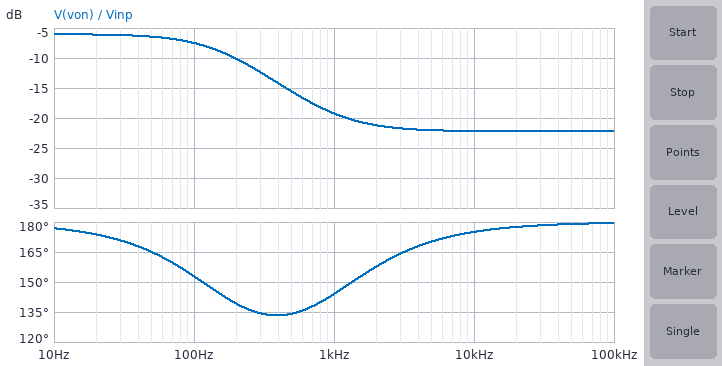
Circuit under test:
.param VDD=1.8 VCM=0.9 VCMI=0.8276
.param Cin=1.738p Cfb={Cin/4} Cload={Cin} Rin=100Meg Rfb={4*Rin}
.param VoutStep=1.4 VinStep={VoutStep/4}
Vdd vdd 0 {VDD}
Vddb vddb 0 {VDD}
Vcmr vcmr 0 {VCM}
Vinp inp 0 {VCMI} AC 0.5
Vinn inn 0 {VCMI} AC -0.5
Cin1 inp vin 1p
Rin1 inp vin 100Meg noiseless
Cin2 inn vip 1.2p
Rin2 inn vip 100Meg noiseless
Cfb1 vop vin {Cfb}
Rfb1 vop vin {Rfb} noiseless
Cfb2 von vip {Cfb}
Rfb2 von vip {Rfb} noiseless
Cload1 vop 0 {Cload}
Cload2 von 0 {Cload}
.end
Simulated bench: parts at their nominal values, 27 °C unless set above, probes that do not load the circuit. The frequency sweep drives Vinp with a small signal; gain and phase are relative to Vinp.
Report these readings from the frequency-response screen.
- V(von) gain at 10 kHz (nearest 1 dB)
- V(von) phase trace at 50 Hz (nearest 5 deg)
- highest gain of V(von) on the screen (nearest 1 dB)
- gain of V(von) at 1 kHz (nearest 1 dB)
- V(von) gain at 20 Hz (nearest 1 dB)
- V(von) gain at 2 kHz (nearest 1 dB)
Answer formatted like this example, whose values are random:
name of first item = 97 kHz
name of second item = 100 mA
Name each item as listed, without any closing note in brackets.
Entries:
V(von) gain at 10 kHz = -22 dB
V(von) phase trace at 50 Hz = 165 deg
highest gain of V(von) on the screen = -6 dB
gain of V(von) at 1 kHz = -19 dB
V(von) gain at 20 Hz = -6 dB
V(von) gain at 2 kHz = -21 dB
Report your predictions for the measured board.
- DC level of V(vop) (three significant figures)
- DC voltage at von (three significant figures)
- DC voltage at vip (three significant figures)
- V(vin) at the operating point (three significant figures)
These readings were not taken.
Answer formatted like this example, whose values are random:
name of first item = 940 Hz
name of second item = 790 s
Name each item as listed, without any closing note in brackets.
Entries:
DC level of V(vop) = 828 mV
DC voltage at von = 828 mV
DC voltage at vip = 828 mV
V(vin) at the operating point = 828 mV
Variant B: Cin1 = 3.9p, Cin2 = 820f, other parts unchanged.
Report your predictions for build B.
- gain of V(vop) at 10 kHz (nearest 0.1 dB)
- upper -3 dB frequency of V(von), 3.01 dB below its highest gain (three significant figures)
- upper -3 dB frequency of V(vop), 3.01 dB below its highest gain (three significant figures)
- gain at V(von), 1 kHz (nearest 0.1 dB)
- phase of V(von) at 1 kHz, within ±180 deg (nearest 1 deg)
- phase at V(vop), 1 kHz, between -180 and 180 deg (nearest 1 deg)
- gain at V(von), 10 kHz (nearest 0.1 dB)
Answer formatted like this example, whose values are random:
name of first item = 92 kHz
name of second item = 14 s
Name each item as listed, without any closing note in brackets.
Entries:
gain of V(vop) at 10 kHz = -14.7 dB
upper -3 dB frequency of V(von), 3.01 dB below its highest gain = 159 Hz
upper -3 dB frequency of V(vop), 3.01 dB below its highest gain = 154 Hz
gain at V(von), 1 kHz = -19.3 dB
phase of V(von) at 1 kHz, within ±180 deg = 142 deg
phase at V(vop), 1 kHz, between -180 and 180 deg = -31 deg
gain at V(von), 10 kHz = -23.0 dB
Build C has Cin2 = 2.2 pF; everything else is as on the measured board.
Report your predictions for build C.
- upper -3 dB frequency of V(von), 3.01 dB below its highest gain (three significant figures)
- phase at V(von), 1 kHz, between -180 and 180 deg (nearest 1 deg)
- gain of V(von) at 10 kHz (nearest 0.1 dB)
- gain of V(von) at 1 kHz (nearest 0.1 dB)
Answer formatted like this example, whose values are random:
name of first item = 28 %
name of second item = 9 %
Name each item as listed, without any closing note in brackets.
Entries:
upper -3 dB frequency of V(von), 3.01 dB below its highest gain = 156 Hz
phase at V(von), 1 kHz, between -180 and 180 deg = 147 deg
gain of V(von) at 10 kHz = -21.2 dB
gain of V(von) at 1 kHz = -18.9 dB
